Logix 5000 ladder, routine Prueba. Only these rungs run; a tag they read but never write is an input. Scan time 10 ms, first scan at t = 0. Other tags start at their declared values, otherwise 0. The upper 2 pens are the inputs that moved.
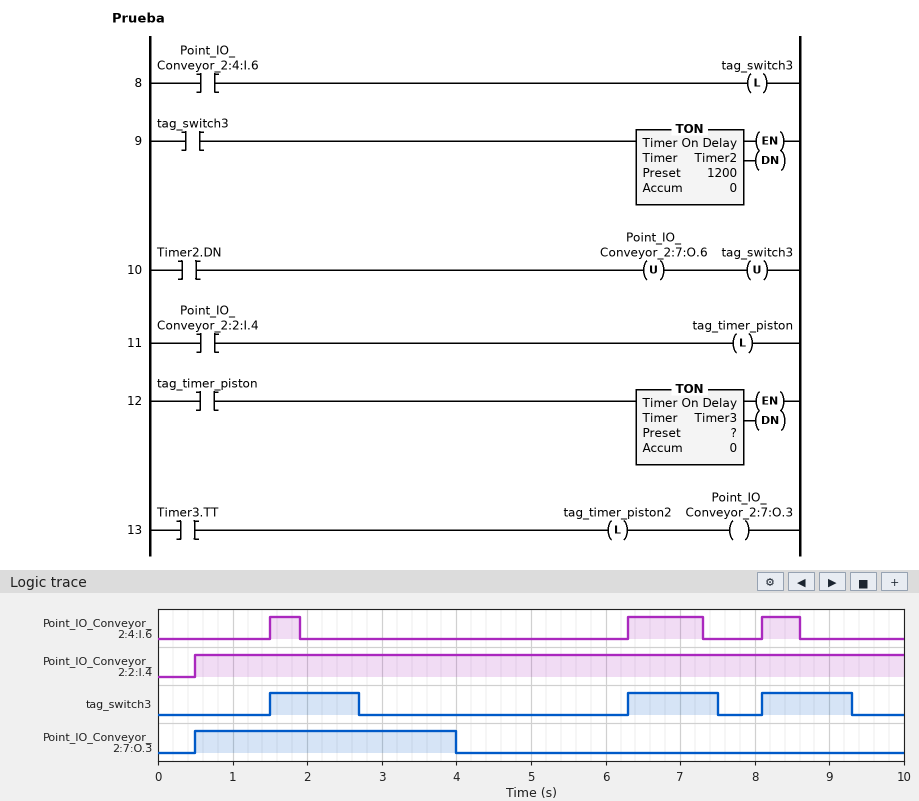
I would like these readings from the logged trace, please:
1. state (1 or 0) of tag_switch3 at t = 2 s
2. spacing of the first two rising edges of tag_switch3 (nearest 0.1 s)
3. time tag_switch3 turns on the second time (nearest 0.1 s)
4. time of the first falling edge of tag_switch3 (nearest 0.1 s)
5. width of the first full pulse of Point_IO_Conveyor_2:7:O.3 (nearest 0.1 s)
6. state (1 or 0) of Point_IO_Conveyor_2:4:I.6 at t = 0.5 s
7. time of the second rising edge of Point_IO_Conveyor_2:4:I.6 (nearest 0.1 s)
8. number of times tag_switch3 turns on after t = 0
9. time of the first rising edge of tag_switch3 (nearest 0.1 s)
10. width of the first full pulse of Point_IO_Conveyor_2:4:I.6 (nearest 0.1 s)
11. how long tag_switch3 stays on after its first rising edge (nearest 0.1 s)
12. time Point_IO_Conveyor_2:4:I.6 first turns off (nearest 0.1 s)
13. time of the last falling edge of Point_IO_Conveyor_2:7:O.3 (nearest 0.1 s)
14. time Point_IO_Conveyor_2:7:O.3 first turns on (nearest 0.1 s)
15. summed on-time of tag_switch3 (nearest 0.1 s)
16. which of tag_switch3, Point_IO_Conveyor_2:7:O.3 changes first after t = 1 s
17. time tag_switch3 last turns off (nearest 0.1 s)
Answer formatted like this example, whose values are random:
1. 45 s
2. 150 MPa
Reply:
1. 1
2. 4.8 s
3. 6.3 s
4. 2.7 s
5. 3.5 s
6. 0
7. 6.3 s
8. 3
9. 1.5 s
10. 0.4 s
11. 1.2 s
12. 1.9 s
13. 4.0 s
14. 0.5 s
15. 3.6 s
16. tag_switch3
17. 9.3 s
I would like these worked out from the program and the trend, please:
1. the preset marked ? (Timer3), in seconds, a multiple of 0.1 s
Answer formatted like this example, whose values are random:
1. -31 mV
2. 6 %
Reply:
1. 3.5 s
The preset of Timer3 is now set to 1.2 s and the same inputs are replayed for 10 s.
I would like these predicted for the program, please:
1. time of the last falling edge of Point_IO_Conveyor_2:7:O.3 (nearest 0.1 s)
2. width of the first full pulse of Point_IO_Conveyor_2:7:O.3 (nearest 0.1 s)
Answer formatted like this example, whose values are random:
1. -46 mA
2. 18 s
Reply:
1. 1.7 s
2. 1.2 s
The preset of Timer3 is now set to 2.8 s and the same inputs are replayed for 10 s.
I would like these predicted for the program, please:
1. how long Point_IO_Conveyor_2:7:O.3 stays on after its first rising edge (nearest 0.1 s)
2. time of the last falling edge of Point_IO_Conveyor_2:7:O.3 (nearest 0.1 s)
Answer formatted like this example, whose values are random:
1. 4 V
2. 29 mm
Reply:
1. 2.8 s
2. 3.3 s
